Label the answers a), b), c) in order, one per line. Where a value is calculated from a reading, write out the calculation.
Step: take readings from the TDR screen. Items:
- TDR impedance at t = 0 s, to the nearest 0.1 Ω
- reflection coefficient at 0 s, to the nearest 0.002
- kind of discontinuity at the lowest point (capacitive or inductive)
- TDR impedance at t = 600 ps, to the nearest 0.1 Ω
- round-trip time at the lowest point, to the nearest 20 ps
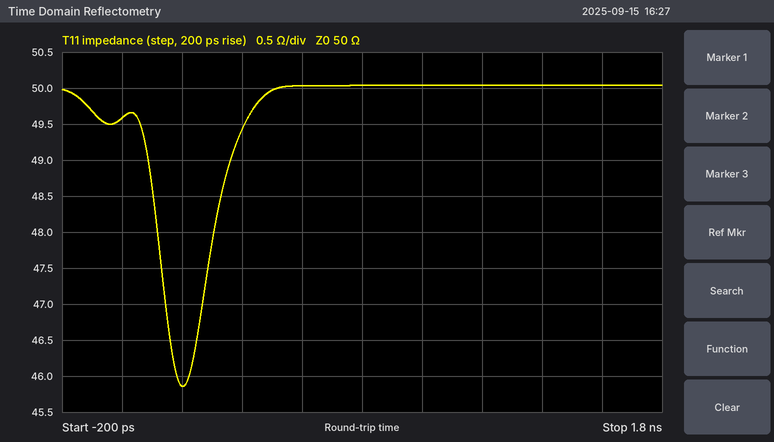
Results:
a) 49.6 Ω
b) (49.6 − 50)/(49.6 + 50) ≈ -0.004
c) capacitive
d) 50.0 Ω
e) 200 ps
